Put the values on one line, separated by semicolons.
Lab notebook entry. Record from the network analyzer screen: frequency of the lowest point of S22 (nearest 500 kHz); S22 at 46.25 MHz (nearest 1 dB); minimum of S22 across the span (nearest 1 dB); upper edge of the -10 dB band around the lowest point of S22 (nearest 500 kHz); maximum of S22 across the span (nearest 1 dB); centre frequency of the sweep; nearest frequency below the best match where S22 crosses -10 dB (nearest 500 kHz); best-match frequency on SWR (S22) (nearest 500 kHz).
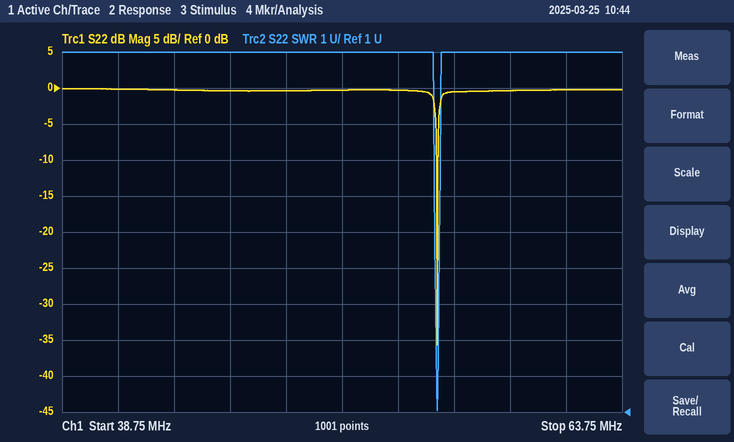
55.5 MHz; 0 dB; -36 dB; 55.5 MHz; 0 dB; 51.25 MHz; 55.5 MHz; 55.5 MHz
